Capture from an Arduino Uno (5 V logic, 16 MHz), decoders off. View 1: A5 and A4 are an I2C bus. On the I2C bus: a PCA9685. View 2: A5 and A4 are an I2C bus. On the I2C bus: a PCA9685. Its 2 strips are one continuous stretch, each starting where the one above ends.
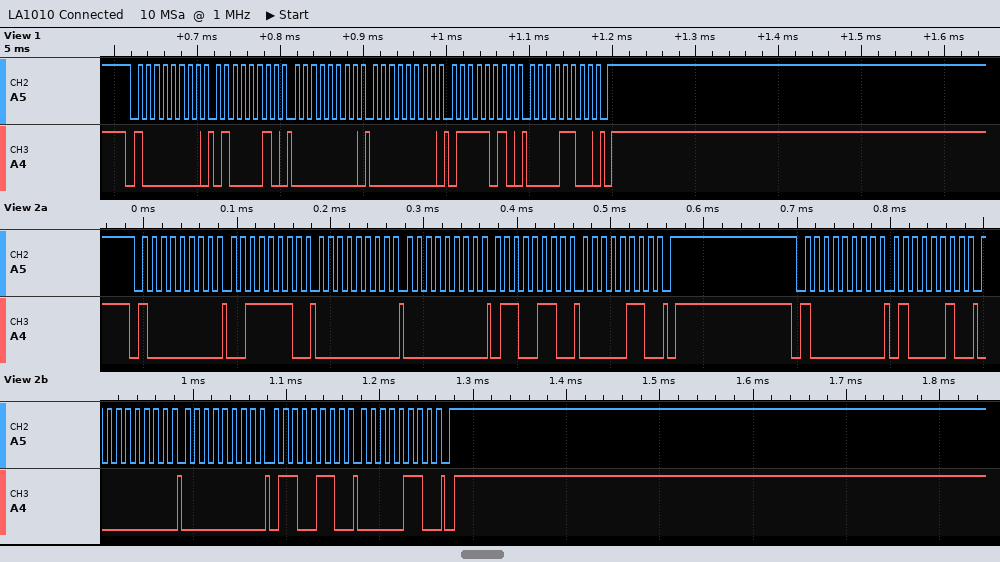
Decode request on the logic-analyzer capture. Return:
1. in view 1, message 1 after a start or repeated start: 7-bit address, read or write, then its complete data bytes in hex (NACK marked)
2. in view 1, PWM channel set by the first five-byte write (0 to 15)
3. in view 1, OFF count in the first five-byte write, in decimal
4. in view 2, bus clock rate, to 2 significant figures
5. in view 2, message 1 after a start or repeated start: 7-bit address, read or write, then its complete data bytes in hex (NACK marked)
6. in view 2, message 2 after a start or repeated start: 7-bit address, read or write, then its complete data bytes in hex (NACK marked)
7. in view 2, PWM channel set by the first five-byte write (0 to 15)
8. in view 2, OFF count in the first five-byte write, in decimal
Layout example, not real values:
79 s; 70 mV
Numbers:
0x40 write: 42 00 00 7A 0C; 15; 3194; 100 kHz; 0x40 write: 3E 00 00 66 06; 0x40 write: 42 00 00 66 06; 14; 1638
